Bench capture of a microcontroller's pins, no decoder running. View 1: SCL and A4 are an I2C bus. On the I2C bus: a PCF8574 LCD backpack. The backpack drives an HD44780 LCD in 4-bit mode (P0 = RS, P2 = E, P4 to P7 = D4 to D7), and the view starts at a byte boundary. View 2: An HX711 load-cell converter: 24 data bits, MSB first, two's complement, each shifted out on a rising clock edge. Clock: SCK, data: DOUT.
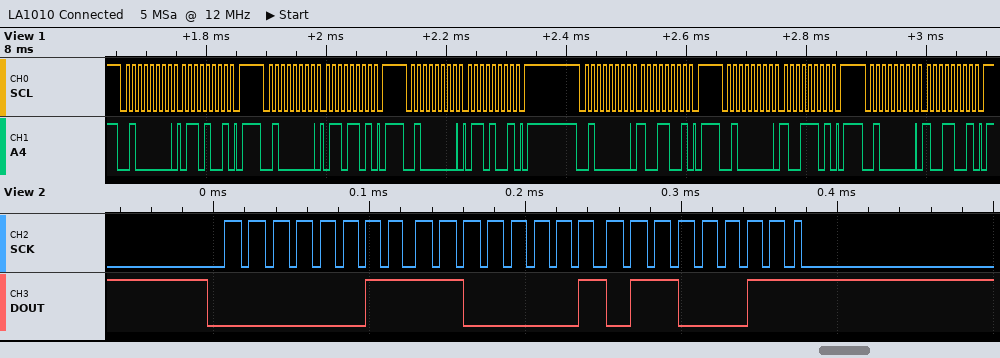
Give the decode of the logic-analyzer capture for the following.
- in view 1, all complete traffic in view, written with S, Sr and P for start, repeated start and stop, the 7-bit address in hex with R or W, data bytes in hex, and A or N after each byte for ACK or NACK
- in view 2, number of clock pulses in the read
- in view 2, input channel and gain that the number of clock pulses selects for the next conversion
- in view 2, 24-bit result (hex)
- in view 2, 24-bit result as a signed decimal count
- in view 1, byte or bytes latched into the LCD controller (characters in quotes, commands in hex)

S 20W A 69 A P S 20W A 6D A P S 20W A 69 A P S 20W A 99 A P S 20W A 9D A P S 20W A 99 A P
25
channel A, gain 128
0x03C163
246115
'i'
